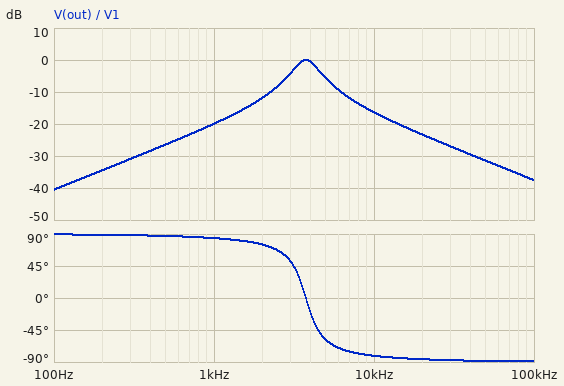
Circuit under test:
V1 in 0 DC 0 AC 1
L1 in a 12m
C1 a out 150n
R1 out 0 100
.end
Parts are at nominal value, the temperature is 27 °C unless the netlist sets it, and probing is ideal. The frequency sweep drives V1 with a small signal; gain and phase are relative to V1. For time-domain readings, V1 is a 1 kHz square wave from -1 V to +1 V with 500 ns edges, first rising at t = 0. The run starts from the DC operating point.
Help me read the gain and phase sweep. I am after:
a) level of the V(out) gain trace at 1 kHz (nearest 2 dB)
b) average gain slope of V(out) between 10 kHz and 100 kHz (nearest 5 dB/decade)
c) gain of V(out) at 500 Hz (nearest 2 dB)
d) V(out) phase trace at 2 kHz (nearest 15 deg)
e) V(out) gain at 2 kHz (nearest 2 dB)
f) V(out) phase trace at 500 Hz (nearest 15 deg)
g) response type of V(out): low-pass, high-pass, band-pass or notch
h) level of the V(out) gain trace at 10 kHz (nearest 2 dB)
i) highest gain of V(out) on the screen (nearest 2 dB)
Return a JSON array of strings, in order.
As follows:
["-20 dB", "-20 dB/decade", "-26 dB", "75 deg", "-12 dB", "90 deg", "band-pass", "-16 dB", "0 dB"]
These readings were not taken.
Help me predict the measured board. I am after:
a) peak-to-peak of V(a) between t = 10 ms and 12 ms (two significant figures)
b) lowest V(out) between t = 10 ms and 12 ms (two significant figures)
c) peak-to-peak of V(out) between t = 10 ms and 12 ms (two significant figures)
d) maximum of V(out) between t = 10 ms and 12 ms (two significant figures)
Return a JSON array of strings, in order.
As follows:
["4.3 V", "-520 mV", "1.0 V", "520 mV"]
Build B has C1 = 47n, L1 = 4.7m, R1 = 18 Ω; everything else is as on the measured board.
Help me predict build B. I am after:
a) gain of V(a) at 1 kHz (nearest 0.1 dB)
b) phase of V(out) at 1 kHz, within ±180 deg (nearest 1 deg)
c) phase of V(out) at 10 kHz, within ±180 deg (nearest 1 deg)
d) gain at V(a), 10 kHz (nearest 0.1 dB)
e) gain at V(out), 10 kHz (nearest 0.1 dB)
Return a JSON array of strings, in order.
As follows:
["0.1 dB", "90 deg", "67 deg", "17.2 dB", "-8.3 dB"]
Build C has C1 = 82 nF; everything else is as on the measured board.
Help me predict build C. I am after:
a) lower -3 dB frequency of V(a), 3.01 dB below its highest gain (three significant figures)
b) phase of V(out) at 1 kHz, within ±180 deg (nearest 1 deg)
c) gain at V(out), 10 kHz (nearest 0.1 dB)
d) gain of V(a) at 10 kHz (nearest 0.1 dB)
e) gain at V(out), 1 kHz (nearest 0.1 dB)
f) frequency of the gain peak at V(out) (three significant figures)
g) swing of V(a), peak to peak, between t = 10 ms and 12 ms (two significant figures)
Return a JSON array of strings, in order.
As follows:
["4.28 kHz", "87 deg", "-15.1 dB", "-8.3 dB", "-25.4 dB", "5.07 kHz", "5.1 V"]
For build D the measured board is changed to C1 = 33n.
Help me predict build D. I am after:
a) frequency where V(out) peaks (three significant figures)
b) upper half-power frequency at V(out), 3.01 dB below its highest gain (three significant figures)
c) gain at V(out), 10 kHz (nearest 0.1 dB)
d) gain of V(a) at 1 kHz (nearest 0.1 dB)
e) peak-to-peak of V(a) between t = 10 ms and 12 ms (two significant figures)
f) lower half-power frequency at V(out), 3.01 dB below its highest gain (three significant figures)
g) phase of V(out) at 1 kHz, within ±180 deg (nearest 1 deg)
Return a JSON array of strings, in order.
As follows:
["8.00 kHz", "8.69 kHz", "-9.2 dB", "0.1 dB", "4.8 V", "7.36 kHz", "89 deg"]
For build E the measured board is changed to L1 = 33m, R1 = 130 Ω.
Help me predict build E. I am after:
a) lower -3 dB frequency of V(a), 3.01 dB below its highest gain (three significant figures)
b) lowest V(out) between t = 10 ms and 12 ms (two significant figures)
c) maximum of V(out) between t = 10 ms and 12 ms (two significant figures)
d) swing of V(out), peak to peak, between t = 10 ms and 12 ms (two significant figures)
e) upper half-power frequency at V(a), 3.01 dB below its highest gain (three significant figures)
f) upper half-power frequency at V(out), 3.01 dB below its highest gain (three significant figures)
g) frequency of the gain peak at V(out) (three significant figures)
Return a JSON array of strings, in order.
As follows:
["1.88 kHz", "-340 mV", "340 mV", "680 mV", "2.52 kHz", "2.60 kHz", "2.26 kHz"]
